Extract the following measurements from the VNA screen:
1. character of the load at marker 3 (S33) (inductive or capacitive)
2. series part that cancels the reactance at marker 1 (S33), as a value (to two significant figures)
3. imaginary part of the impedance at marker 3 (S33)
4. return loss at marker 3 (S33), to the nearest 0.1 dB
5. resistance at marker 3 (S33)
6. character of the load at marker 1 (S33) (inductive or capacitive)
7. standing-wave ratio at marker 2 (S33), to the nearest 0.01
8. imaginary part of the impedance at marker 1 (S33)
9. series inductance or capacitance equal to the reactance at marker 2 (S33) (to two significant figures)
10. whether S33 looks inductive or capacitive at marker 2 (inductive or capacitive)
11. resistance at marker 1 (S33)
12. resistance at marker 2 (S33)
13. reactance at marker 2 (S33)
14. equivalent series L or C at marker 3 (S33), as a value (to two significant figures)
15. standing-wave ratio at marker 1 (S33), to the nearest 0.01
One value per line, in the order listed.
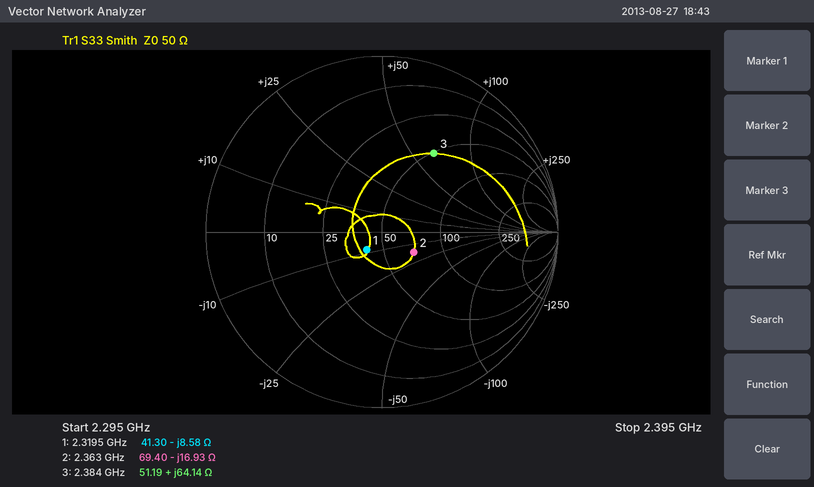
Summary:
inductive
590 pH
+64.14 Ω
5.4 dB
51.19 Ω
capacitive
1.54
-8.58 Ω
4.0 pF
capacitive
41.30 Ω
69.40 Ω
-16.93 Ω
4.3 nH
1.31
